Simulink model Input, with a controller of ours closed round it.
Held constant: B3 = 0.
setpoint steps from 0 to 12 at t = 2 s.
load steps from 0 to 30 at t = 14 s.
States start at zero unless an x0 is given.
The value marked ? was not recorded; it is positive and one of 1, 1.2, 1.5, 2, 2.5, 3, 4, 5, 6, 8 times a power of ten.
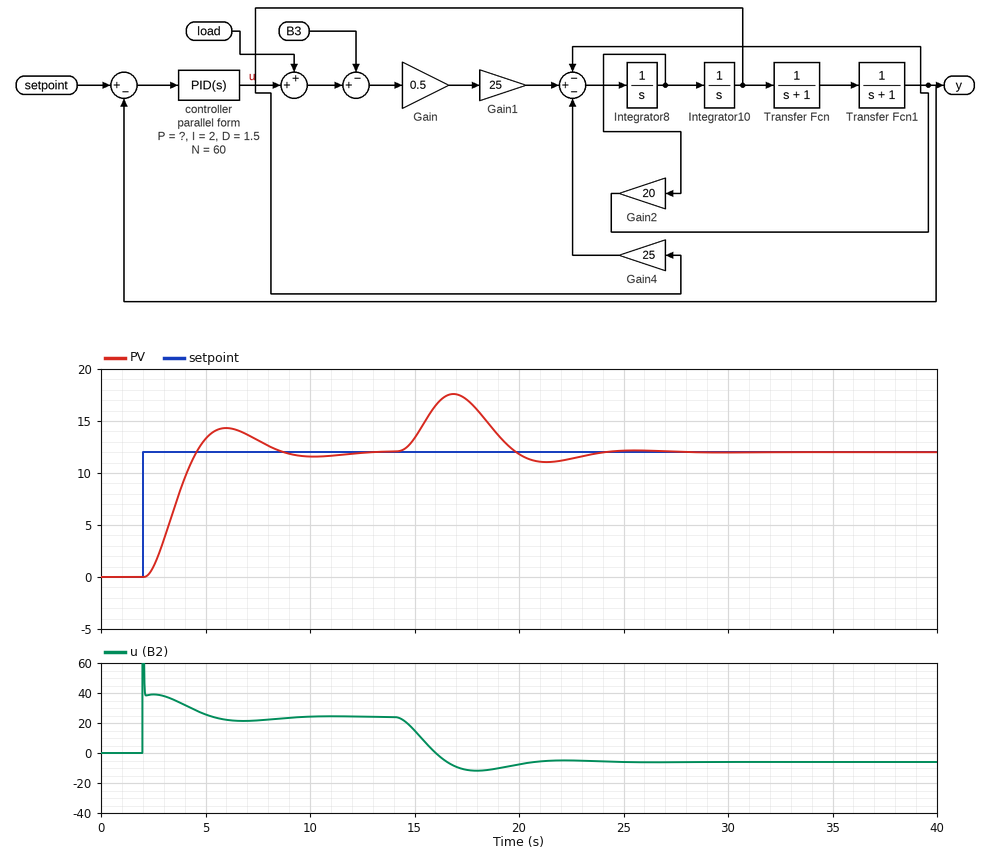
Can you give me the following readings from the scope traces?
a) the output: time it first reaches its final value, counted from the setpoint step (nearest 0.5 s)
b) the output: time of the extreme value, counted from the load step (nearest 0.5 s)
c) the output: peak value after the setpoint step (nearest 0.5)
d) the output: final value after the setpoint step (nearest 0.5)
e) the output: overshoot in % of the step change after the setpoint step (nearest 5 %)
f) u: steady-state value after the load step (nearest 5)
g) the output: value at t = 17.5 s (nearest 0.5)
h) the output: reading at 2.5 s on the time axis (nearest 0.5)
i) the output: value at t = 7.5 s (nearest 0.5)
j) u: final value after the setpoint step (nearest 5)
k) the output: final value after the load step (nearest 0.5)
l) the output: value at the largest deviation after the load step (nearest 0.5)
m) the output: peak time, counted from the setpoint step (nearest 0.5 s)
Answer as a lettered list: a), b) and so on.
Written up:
a) 2.5 s
b) 3.0 s
c) 14.5
d) 12.0
e) 20 %
f) -5
g) 17.0
h) 1.0
i) 13.0
j) 25
k) 12.0
l) 17.5
m) 4.0 s
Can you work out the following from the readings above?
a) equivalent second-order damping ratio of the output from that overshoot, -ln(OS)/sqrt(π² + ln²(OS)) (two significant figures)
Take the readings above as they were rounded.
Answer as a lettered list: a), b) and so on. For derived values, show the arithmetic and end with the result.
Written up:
a) ln(0.2) = -1.609; 1.609 / sqrt(9.870 + 2.590) = 0.46
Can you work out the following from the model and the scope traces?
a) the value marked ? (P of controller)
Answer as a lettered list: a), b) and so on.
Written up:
a) 3
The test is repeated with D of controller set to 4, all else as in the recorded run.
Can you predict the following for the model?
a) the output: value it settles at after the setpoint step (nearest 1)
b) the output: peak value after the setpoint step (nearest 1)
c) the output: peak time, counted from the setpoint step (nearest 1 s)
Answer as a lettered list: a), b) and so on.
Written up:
a) 12
b) 13
c) 6 s
